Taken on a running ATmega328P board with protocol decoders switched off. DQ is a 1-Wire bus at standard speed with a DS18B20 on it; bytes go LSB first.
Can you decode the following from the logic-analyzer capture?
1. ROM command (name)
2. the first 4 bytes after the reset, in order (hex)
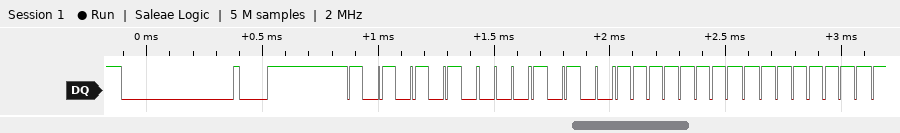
Match ROM
55 28 FF FF
